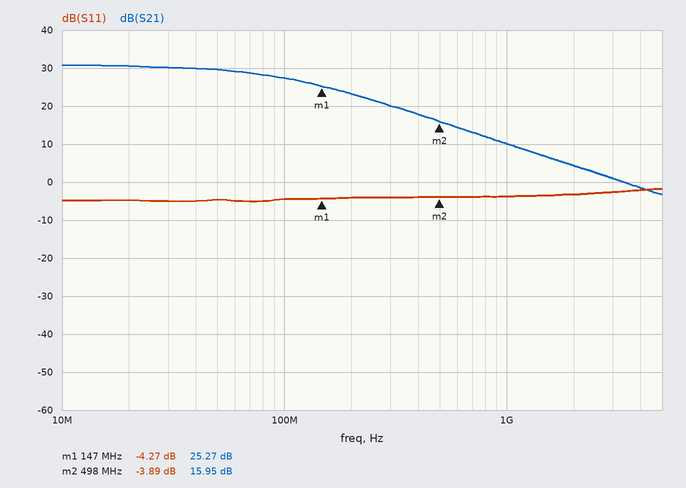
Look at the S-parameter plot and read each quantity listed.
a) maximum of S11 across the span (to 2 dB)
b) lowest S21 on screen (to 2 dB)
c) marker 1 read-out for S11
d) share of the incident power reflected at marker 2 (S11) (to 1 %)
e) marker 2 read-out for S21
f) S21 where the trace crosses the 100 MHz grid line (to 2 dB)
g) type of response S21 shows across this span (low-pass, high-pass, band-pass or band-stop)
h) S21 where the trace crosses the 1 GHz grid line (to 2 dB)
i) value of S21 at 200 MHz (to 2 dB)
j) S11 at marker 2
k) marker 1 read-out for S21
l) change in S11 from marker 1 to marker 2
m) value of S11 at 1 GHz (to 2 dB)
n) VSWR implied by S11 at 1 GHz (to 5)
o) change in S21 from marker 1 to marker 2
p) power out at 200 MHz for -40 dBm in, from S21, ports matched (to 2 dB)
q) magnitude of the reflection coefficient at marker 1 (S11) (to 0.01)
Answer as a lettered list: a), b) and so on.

a) -2 dB
b) -4 dB
c) -4.27 dB
d) 41 %
e) 15.95 dB
f) 28 dB
g) low-pass
h) 10 dB
i) 24 dB
j) -3.89 dB
k) 25.27 dB
l) 0.38 dB
m) -4 dB
n) 5
o) -9.32 dB
p) -16 dBm
q) 0.61
